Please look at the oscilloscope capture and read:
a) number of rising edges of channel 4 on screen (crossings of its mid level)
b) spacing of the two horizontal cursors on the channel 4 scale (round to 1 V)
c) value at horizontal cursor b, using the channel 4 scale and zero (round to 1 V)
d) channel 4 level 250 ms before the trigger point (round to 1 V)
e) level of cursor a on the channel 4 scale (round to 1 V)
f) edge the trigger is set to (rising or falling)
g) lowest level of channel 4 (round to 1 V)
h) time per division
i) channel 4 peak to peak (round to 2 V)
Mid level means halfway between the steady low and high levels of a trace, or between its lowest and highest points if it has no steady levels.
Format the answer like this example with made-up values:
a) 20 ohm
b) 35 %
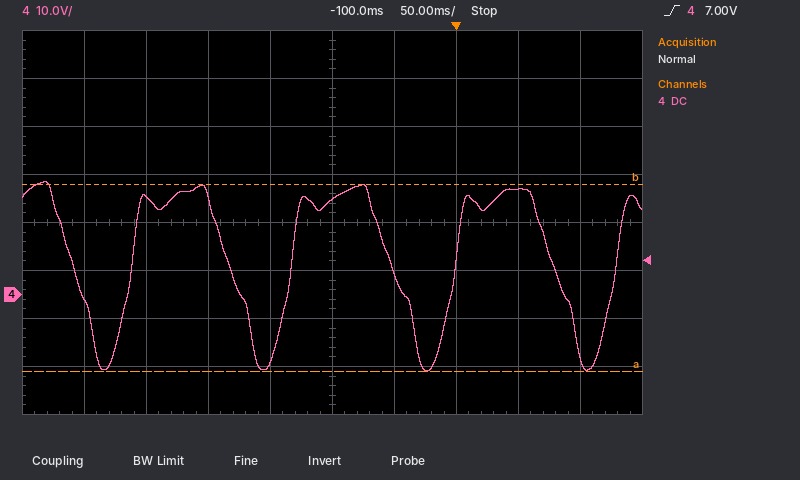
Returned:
a) 4
b) 39 V
c) 23 V
d) 20 V
e) -16 V
f) rising
g) -16 V
h) 50 ms
i) 40 V
